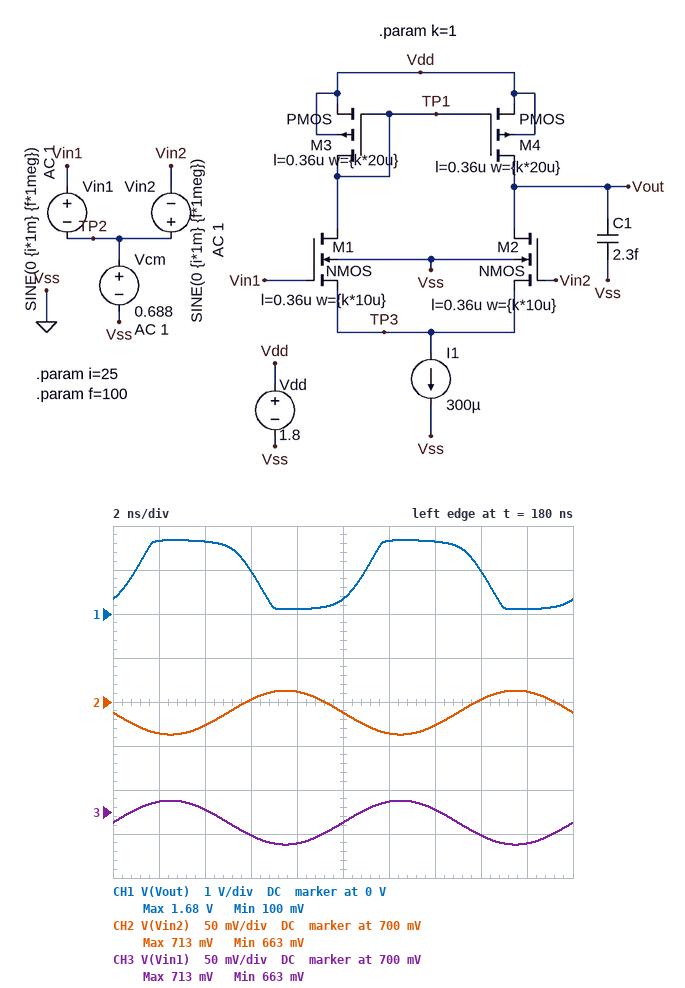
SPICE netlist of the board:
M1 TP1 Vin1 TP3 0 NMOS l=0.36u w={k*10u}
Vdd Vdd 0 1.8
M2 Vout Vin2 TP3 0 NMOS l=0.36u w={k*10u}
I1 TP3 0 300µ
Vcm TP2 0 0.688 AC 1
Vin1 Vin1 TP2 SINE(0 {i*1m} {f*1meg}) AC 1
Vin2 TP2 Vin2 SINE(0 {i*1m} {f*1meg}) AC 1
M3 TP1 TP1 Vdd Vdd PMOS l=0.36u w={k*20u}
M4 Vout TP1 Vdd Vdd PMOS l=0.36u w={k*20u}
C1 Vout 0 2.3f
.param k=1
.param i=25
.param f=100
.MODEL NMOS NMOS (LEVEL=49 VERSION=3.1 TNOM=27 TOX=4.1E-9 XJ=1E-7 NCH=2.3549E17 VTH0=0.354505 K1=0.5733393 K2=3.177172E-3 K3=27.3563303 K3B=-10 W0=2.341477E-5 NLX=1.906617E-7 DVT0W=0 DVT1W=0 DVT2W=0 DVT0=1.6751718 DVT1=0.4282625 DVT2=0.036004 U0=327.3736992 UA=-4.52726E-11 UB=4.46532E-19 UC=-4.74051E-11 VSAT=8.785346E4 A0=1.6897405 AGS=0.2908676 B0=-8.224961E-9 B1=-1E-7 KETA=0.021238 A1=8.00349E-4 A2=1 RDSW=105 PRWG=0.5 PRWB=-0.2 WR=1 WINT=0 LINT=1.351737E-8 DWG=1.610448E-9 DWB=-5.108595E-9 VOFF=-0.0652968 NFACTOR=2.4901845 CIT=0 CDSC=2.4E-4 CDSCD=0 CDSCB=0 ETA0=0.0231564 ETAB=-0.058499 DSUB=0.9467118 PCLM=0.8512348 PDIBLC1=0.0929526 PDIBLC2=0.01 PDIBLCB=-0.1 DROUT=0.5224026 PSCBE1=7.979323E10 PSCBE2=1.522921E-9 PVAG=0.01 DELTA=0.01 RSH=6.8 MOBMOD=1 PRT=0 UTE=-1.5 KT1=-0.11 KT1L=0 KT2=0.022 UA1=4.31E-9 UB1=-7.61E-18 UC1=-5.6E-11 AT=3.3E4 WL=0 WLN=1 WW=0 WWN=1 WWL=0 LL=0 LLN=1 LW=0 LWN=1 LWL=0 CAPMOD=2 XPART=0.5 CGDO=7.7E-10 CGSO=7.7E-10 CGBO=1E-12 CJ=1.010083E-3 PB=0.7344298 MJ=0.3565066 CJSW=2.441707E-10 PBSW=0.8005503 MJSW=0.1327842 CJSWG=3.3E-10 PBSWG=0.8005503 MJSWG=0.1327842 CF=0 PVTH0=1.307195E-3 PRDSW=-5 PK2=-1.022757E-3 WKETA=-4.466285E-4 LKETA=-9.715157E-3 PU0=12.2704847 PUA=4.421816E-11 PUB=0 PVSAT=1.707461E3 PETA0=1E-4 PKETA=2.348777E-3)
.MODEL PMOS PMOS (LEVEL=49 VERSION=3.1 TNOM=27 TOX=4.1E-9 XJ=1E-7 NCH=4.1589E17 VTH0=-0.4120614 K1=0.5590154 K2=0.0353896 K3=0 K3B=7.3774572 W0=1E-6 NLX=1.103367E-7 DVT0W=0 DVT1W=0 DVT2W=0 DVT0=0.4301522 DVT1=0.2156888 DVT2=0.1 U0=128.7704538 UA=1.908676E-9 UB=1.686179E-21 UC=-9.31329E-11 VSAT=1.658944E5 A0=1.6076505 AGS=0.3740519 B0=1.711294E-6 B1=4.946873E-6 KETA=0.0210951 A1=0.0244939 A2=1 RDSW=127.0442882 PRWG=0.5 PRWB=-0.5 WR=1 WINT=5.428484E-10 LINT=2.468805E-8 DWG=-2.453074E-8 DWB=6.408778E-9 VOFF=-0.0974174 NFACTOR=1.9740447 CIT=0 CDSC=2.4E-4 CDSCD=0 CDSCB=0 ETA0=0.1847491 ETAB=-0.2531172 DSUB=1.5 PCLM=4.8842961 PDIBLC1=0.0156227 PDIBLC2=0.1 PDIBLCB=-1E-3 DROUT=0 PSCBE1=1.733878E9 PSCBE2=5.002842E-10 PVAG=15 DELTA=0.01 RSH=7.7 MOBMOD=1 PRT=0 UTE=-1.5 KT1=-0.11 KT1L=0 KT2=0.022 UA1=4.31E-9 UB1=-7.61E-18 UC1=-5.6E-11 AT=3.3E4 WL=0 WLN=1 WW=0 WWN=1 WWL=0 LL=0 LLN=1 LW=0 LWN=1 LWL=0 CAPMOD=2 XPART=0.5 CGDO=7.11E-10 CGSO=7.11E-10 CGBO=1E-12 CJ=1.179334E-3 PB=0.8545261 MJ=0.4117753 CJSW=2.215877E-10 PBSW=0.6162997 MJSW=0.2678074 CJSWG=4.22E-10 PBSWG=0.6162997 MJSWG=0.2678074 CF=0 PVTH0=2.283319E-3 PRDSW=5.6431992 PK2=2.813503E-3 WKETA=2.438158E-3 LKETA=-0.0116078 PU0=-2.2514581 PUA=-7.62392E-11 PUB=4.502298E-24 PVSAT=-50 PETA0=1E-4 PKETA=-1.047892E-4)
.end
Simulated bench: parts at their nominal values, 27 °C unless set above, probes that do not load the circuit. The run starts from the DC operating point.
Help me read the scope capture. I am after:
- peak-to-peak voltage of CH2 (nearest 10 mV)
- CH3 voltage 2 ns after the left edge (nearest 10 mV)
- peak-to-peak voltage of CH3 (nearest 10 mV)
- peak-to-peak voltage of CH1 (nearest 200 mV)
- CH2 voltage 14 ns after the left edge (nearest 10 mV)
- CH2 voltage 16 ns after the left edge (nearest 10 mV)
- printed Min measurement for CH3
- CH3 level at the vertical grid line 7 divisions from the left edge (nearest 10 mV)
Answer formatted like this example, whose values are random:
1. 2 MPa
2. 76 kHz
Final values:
1. 50 mV
2. 710 mV
3. 50 mV
4. 1.6 V
5. 670 mV
6. 700 mV
7. 663 mV
8. 700 mV
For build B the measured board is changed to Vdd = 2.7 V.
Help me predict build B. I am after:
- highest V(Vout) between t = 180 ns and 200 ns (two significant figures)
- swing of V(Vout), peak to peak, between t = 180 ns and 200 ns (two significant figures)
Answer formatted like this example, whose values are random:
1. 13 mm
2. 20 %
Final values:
1. 2.6 V
2. 2.4 V
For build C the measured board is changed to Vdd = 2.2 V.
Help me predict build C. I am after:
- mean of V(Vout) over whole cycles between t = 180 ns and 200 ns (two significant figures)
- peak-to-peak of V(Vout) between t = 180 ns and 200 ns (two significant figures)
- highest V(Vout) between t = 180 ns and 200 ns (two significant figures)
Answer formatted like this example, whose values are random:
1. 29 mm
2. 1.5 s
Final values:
1. 1.2 V
2. 2.0 V
3. 2.1 V
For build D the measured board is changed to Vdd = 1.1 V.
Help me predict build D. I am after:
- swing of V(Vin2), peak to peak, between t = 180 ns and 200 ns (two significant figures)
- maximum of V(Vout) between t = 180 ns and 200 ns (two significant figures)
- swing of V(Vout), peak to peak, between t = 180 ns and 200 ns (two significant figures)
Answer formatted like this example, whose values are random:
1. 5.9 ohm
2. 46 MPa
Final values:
1. 50 mV
2. 970 mV
3. 890 mV
